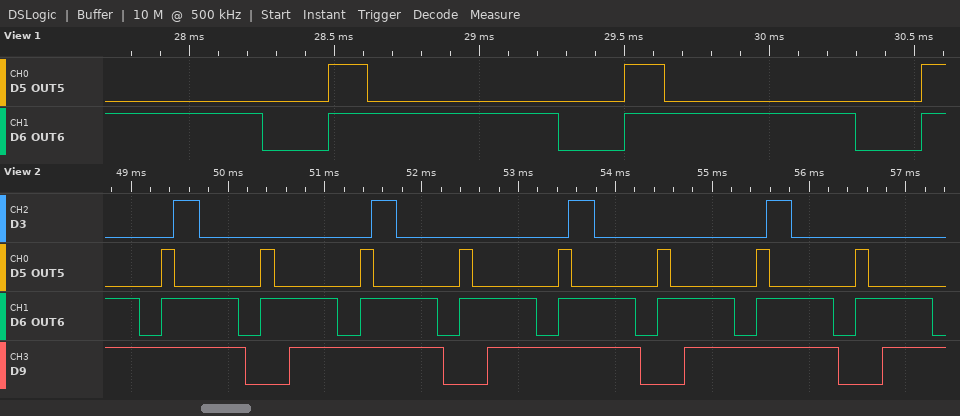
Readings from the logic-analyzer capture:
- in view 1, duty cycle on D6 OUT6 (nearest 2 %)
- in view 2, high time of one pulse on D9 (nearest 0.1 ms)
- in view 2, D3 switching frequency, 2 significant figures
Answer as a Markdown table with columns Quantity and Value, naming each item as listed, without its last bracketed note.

| Quantity | Value |
|---|---|
| in view 1, duty cycle on D6 OUT6 | 78 % |
| in view 2, high time of one pulse on D9 | 1.6 ms |
| in view 2, D3 switching frequency, 2 significant figures | 490 Hz |
